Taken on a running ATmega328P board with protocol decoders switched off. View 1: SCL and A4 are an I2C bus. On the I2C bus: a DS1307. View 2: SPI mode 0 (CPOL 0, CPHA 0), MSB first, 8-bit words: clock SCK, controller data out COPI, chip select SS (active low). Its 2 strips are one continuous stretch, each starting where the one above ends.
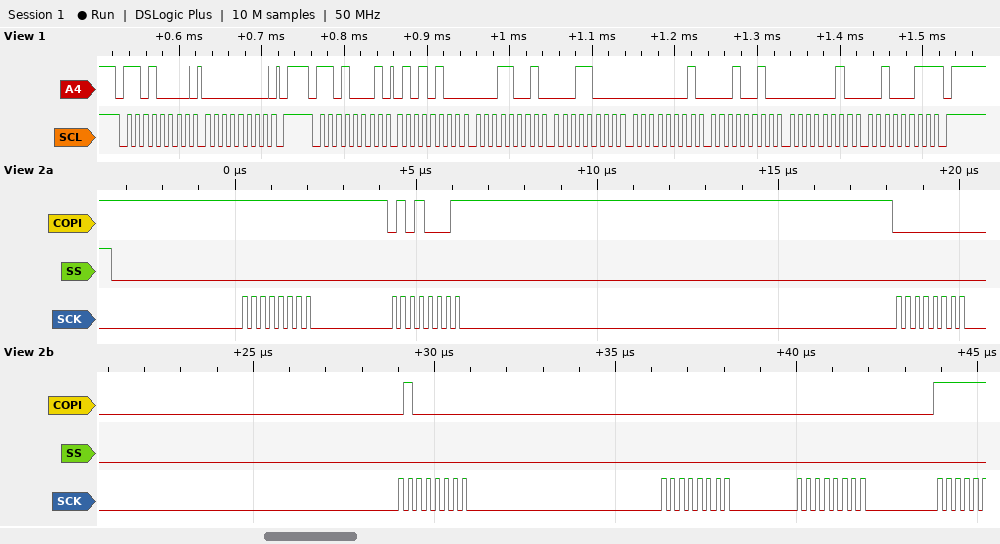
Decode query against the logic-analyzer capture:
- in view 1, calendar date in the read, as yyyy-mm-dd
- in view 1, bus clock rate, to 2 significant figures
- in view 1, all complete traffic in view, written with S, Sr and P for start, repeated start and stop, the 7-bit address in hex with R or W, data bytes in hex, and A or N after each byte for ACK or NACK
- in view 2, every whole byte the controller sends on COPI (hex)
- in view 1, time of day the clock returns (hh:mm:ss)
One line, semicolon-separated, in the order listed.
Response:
2023-02-12; 100 kHz; S 68W A 00 A P S 68R A 54 A 19 A 18 A 01 A 12 A 02 A 23 N P; FF 51 00 40 00 00; 18:19:54
